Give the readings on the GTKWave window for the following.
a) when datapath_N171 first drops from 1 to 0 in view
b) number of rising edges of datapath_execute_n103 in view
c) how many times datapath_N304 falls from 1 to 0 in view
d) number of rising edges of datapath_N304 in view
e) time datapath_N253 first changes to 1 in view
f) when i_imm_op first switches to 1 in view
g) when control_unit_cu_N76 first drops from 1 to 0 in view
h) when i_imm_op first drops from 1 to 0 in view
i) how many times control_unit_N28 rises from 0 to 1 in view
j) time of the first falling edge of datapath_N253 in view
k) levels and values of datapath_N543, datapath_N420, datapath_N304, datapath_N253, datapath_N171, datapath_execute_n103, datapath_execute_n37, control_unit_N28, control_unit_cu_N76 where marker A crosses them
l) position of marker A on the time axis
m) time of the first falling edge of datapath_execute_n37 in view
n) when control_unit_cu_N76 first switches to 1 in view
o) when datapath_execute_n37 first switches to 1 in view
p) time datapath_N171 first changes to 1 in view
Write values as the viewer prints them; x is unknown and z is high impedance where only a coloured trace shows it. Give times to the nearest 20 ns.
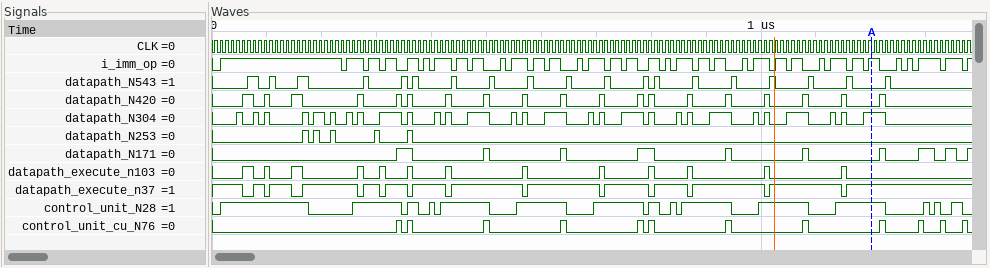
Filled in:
360 ns
13
29
29
160 ns
20 ns
340 ns
240 ns
15
180 ns
datapath_N543=0, datapath_N420=0, datapath_N304=1, datapath_N253=0, datapath_N171=0, datapath_execute_n103=0, datapath_execute_n37=1, control_unit_N28=1, control_unit_cu_N76=0
1200 ns
60 ns
340 ns
80 ns
340 ns
